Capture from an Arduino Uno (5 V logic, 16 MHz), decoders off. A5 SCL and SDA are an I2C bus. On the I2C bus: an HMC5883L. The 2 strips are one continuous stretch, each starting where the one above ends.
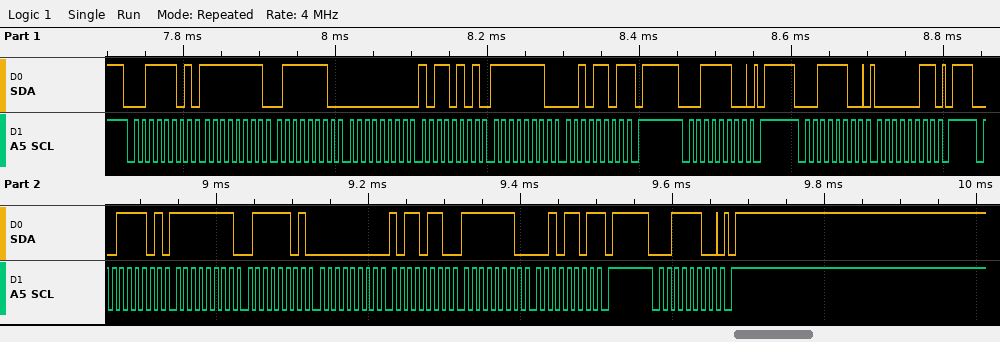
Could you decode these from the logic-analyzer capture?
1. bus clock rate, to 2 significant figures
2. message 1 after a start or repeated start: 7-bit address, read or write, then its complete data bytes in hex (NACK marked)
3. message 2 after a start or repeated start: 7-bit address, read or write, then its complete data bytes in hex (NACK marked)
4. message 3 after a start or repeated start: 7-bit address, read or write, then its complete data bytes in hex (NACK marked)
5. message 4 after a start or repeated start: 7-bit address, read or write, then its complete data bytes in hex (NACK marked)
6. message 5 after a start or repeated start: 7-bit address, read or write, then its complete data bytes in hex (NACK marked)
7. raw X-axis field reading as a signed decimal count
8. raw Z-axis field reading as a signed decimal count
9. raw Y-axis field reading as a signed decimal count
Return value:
100 kHz
0x1E read: FF 7E 00 B5 FE 2D NACK
0x1E write
0x1E write: 03
0x1E read: FF 7D 00 B6 FE 2D NACK
0x1E write
-131
182
-467
